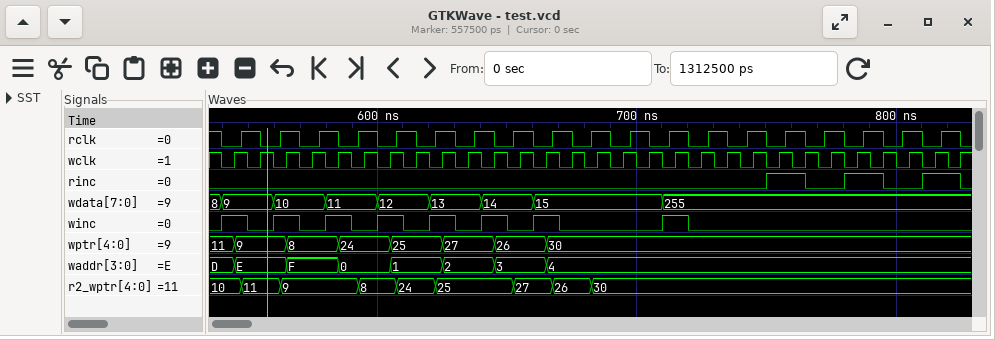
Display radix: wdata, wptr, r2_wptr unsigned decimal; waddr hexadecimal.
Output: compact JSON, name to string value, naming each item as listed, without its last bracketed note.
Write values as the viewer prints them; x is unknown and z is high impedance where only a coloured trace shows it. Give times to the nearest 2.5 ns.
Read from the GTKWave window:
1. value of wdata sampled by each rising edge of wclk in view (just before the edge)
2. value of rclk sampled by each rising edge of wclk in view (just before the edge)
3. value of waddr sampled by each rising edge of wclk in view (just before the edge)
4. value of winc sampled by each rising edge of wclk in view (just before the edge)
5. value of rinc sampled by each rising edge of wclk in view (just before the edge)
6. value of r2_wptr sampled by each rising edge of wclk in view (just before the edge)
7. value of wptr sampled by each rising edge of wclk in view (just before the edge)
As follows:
{"value of wdata sampled by each rising edge of wclk in view": "9, 9, 10, 10, 11, 11, 12, 12, 13, 13, 14, 14, 15, 15, 15, 15, 15, 255, 255, 255, 255, 255, 255, 255, 255, 255, 255, 255, 255", "value of rclk sampled by each rising edge of wclk in view": "0 1 1 0 1 1 0 1 1 0 1 1 0 1 1 0 1 1 0 1 1 0 1 1 0 1 1 0 1", "value of waddr sampled by each rising edge of wclk in view": "D, E, E, F, F, 0, 0, 1, 1, 2, 2, 3, 3, 4, 4, 4, 4, 4, 4, 4, 4, 4, 4, 4, 4, 4, 4, 4, 4", "value of winc sampled by each rising edge of wclk in view": "1 0 1 0 1 0 1 0 1 0 1 0 1 0 0 0 0 1 0 0 0 0 0 0 0 0 0 0 0", "value of rinc sampled by each rising edge of wclk in view": "0 0 0 0 0 0 0 0 0 0 0 0 0 0 0 0 0 0 0 0 0 1 1 0 1 1 0 1 1", "value of r2_wptr sampled by each rising edge of wclk in view": "10, 11, 9, 9, 9, 8, 8, 24, 25, 25, 25, 27, 27, 26, 30, 30, 30, 30, 30, 30, 30, 30, 30, 30, 30, 30, 30, 30, 30", "value of wptr sampled by each rising edge of wclk in view": "11, 9, 9, 8, 8, 24, 24, 25, 25, 27, 27, 26, 26, 30, 30, 30, 30, 30, 30, 30, 30, 30, 30, 30, 30, 30, 30, 30, 30"}
